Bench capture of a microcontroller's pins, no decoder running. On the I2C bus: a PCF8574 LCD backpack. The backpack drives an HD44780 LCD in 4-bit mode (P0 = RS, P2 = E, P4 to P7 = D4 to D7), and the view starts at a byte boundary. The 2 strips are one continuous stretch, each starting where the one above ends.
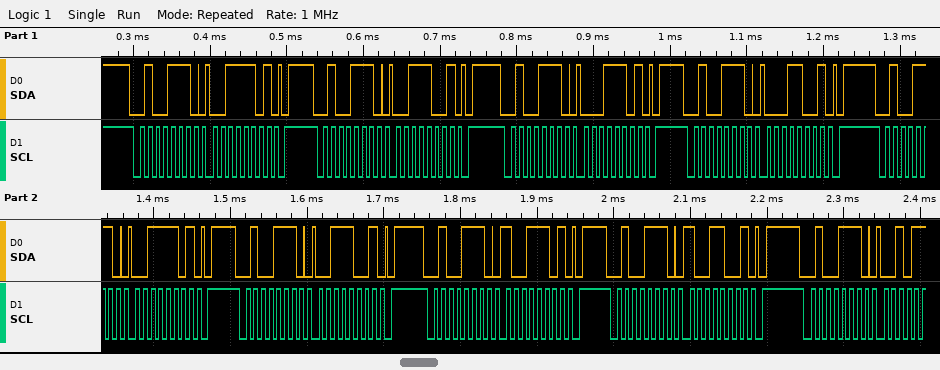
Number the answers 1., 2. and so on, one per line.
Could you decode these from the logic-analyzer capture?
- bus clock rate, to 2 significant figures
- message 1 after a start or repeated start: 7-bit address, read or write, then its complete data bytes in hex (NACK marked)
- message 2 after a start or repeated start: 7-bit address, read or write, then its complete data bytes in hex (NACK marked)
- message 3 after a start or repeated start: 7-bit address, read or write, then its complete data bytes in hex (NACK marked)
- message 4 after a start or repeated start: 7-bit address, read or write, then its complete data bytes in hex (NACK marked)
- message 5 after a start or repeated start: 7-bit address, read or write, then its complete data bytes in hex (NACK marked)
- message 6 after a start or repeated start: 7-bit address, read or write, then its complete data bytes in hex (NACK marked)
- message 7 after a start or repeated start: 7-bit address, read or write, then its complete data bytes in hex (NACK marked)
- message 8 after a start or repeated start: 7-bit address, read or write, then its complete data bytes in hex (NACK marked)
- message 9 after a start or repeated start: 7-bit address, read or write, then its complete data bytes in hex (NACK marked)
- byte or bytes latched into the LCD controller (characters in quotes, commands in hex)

1. 100 kHz
2. 0x27 write: 3D
3. 0x27 write: 39
4. 0x27 write: 1D
5. 0x27 write: 19
6. 0x27 write: 3D
7. 0x27 write: 39
8. 0x27 write: 9D
9. 0x27 write: 99
10. 0x27 write
11. '1' '9'
